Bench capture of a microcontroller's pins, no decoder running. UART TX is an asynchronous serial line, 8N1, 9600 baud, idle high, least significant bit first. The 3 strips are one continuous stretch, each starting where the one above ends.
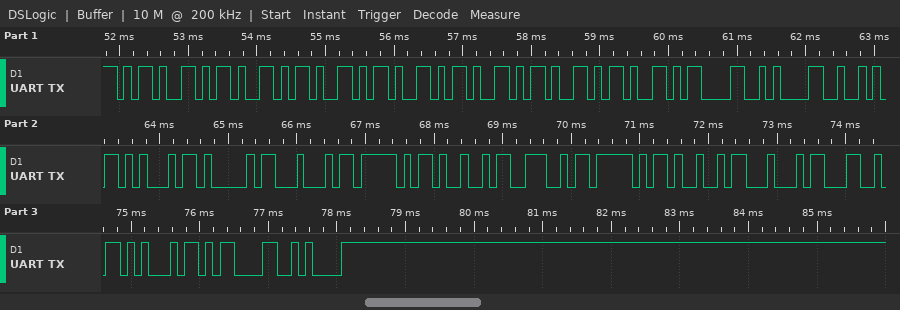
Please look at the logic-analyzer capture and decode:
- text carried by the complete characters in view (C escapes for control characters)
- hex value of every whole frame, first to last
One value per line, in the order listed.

"-------\r\nREAD_IN_IDLE\r\n"
2D 2D 2D 2D 2D 2D 2D 0D 0A 52 45 41 44 5F 49 4E 5F 49 44 4C 45 0D 0A
